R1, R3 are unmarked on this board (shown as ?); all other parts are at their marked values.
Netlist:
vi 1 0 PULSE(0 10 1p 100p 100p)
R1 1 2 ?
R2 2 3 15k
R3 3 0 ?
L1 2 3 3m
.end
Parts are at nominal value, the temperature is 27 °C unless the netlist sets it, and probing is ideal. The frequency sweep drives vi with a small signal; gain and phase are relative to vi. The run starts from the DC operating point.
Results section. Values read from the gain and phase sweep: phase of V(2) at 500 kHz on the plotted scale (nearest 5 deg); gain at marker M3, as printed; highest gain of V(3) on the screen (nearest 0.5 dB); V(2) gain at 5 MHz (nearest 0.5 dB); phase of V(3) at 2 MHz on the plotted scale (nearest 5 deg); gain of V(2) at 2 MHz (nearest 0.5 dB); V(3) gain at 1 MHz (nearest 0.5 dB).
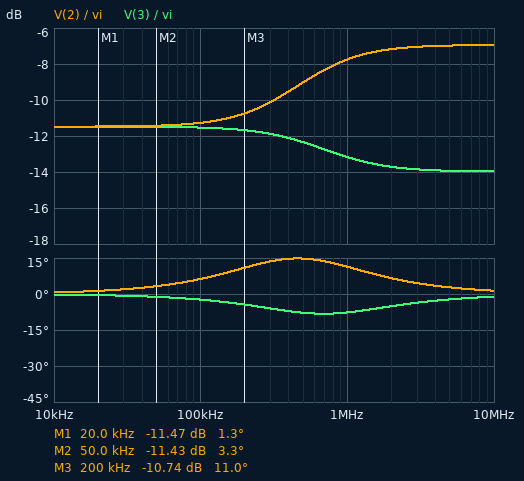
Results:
15 deg
-10.74 dB
-11.5 dB
-7.0 dB
-5 deg
-7.0 dB
-13.0 dB
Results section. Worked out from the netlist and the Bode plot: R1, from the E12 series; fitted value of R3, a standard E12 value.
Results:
33 kΩ
12 kΩ
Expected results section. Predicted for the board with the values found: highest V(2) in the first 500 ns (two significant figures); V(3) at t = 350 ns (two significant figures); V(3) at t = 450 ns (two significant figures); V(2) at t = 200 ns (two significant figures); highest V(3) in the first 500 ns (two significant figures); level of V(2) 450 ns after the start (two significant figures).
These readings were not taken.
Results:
4.5 V
2.5 V
2.5 V
3.5 V
2.6 V
3.0 V
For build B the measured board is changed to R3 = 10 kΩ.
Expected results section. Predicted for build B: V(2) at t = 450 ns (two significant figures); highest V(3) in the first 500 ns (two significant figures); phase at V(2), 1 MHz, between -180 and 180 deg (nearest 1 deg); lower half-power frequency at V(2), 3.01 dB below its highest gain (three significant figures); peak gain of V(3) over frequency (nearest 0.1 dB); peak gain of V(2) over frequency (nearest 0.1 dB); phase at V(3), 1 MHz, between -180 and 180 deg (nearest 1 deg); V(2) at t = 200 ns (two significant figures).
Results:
2.7 V
2.2 V
13 deg
381 kHz
-12.7 dB
-7.3 dB
-8 deg
3.3 V
